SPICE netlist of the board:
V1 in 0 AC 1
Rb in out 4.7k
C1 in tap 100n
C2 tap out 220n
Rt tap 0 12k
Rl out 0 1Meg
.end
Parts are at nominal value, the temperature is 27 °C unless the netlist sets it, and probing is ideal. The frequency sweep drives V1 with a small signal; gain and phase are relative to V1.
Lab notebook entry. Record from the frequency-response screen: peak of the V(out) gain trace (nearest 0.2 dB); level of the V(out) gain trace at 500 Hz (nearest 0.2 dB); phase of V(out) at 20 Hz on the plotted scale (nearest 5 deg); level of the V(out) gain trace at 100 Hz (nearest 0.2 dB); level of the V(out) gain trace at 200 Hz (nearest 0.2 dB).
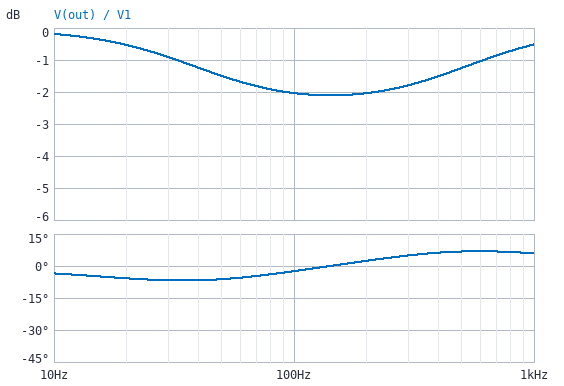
-0.2 dB
-1.2 dB
-5 deg
-2.0 dB
-2.0 dB
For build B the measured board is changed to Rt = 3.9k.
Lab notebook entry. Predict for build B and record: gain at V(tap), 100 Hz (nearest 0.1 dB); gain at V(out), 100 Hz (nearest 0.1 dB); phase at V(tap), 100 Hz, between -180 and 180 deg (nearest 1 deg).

-6.4 dB
-3.2 dB
42 deg
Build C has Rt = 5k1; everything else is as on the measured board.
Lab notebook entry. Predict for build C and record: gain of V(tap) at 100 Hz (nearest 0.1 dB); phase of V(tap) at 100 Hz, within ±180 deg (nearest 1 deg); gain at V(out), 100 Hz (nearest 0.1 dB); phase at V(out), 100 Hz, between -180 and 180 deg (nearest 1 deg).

-5.0 dB
37 deg
-3.1 dB
-12 deg
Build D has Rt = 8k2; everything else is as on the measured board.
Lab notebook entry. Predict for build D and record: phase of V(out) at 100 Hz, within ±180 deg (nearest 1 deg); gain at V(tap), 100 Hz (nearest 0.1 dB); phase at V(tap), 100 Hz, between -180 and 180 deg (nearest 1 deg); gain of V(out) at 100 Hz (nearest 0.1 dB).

-6 deg
-3.1 dB
28 deg
-2.6 dB
